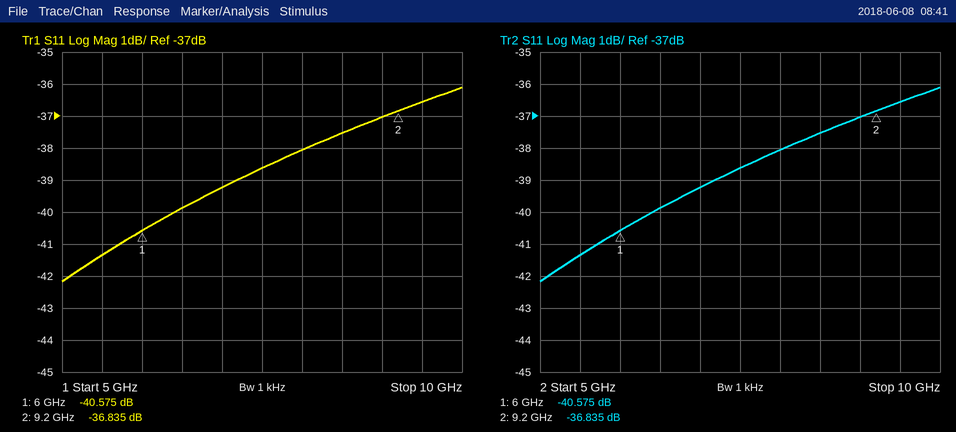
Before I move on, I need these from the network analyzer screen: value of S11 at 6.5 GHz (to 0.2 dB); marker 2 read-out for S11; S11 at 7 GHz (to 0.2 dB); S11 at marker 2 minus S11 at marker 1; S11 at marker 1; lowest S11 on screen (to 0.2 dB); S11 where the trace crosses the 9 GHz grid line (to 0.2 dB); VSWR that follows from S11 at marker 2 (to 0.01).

-39.8 dB
-36.835 dB
-39.2 dB
3.740 dB
-40.575 dB
-42.2 dB
-37.0 dB
1.03
